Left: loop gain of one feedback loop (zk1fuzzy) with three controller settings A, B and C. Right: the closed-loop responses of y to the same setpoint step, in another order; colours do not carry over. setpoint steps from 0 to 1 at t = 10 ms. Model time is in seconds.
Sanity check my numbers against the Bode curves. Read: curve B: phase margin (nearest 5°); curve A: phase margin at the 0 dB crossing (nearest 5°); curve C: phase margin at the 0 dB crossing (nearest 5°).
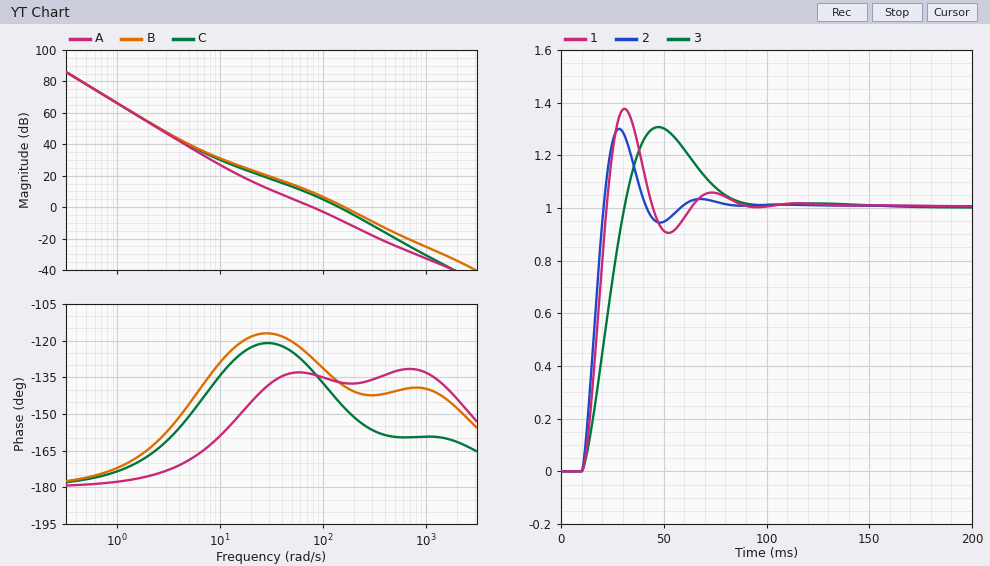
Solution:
40°
45°
35°
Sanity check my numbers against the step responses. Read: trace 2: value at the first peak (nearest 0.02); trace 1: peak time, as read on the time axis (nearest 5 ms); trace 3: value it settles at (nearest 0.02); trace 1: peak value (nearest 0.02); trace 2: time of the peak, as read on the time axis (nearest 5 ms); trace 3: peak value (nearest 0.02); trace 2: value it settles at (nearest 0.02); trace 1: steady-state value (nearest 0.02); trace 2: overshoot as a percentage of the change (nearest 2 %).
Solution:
1.30
30 ms
1.00
1.38
30 ms
1.30
1.00
1.00
30 %
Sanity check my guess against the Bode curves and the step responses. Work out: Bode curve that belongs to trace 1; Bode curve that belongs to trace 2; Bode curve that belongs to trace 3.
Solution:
C
B
A
